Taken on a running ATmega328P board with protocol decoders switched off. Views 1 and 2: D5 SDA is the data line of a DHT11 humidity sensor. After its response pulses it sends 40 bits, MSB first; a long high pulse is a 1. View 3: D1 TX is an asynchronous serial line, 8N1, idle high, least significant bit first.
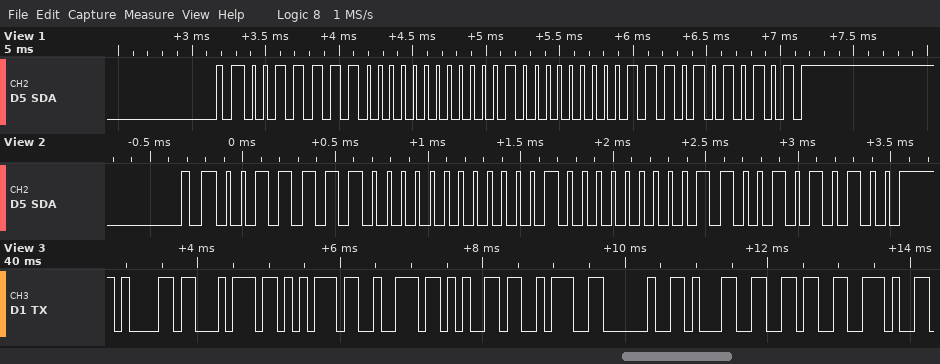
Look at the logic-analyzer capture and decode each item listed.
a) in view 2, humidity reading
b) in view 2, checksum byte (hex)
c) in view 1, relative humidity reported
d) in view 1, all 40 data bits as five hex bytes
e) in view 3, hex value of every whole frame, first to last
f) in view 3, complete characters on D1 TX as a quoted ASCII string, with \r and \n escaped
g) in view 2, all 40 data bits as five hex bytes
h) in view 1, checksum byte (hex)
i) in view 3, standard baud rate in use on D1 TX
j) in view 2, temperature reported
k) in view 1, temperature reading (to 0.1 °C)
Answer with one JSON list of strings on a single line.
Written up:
["62 %", "0x54", "62 %", "3E 00 10 07 55", "0x61 0x74 0x75 0x72 0x65 0x3A 0x20 0x31 0x36 0x2E", "\"ature: 16.\"", "3E 00 10 06 54", "0x55", "9600 baud", "16.6 °C", "16.7 °C"]
